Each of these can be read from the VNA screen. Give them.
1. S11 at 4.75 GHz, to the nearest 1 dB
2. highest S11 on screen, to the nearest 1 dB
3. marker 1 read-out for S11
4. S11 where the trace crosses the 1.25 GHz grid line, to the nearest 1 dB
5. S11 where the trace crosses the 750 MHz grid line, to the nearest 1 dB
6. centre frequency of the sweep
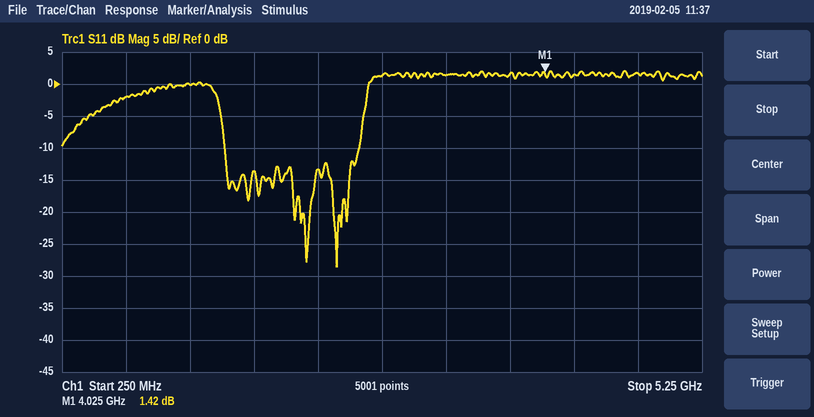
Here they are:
2 dB
2 dB
1.42 dB
0 dB
-2 dB
2.75 GHz
